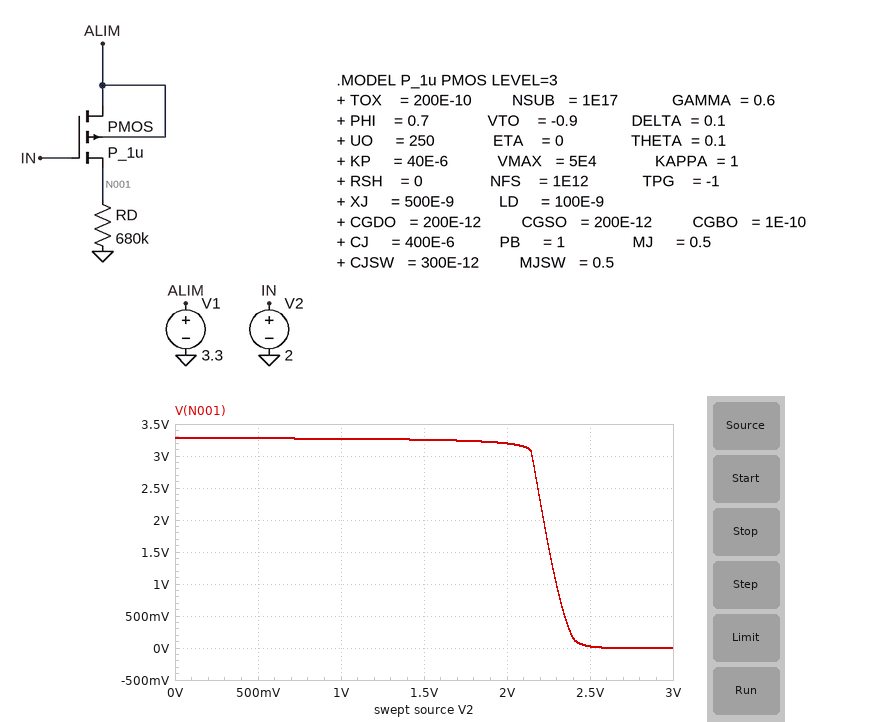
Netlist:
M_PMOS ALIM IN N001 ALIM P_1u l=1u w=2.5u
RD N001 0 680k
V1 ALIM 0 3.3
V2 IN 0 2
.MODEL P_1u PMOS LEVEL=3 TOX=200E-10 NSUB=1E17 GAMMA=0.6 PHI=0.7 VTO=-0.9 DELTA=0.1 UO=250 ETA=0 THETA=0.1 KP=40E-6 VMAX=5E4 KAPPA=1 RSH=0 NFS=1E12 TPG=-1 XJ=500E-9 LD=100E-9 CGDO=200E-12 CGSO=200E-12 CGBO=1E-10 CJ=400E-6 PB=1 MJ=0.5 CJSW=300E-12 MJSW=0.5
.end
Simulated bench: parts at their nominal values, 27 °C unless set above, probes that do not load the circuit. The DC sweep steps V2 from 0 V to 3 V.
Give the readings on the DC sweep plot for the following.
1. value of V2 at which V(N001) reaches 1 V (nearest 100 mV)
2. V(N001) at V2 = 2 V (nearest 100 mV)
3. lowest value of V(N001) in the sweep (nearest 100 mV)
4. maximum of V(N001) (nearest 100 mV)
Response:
2.3 V
3.2 V
0 V
3.3 V
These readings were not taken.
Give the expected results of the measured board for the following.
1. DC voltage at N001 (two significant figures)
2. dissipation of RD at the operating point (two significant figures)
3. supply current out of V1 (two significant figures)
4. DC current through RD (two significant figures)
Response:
3.2 V
15 µW
4.7 µA
4.7 µA
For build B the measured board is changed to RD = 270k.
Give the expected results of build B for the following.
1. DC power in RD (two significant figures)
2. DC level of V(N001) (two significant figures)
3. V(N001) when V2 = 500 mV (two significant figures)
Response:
24 µW
2.5 V
3.2 V
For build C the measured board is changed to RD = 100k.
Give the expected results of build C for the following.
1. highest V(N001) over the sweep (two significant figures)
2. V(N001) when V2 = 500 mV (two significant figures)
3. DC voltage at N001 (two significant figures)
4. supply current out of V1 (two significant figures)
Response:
3.2 V
3.1 V
1.0 V
10 µA
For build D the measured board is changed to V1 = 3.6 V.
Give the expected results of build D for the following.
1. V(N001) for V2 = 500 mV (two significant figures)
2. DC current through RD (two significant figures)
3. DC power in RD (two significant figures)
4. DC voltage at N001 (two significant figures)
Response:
3.6 V
5.2 µA
18 µW
3.5 V
